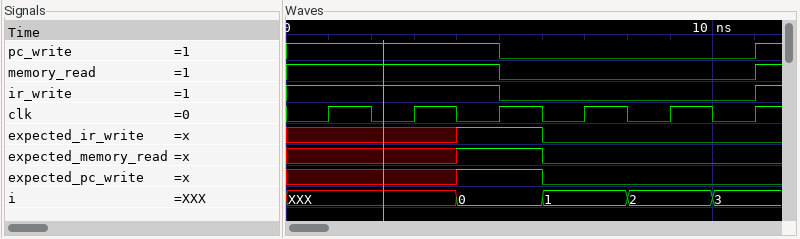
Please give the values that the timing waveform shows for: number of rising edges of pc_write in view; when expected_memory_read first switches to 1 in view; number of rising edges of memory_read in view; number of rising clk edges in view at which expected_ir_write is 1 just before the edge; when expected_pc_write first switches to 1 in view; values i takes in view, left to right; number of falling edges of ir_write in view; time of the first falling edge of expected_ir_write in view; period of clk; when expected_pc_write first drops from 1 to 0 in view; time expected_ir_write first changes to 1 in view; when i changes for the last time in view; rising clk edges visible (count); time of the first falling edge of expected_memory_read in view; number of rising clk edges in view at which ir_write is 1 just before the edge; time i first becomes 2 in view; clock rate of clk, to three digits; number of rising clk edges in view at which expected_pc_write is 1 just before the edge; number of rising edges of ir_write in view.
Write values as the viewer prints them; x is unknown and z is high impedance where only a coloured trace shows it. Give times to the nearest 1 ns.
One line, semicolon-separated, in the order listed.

1; 4 ns; 1; 1; 4 ns; XXX, 0, 1, 2, 3; 1; 6 ns; 2 ns; 6 ns; 4 ns; 10 ns; 6; 6 ns; 3; 8 ns; 500 MHz; 1; 1
